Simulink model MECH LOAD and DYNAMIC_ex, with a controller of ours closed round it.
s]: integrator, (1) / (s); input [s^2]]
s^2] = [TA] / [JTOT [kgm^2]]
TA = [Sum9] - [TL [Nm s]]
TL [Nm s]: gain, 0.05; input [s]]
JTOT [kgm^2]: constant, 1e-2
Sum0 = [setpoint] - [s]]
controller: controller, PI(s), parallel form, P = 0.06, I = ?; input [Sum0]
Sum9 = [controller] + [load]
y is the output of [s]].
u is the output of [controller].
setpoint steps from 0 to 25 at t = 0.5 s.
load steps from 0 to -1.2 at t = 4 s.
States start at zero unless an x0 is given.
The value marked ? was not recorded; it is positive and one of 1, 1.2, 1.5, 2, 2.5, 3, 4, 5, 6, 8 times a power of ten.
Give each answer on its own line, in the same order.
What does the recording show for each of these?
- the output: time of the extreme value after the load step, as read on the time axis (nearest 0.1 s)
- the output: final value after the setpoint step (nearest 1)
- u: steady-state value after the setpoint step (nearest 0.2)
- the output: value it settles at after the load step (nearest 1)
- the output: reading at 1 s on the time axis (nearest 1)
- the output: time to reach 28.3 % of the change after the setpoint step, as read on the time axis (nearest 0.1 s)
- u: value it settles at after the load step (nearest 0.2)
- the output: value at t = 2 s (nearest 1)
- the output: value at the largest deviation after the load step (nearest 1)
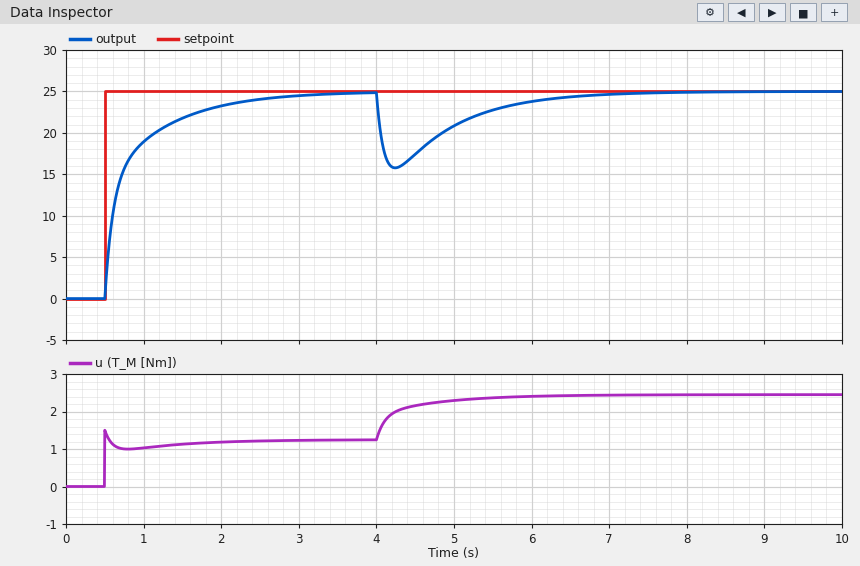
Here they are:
4.2 s
25
1.2
25
19
0.6 s
2.4
23
16
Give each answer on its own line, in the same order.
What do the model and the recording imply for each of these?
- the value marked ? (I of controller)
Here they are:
0.12
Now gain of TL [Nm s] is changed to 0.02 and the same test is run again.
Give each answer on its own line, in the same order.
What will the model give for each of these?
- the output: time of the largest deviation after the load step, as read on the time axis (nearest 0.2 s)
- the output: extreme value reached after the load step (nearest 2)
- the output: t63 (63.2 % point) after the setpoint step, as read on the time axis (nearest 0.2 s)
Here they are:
4.2 s
14
0.6 s
